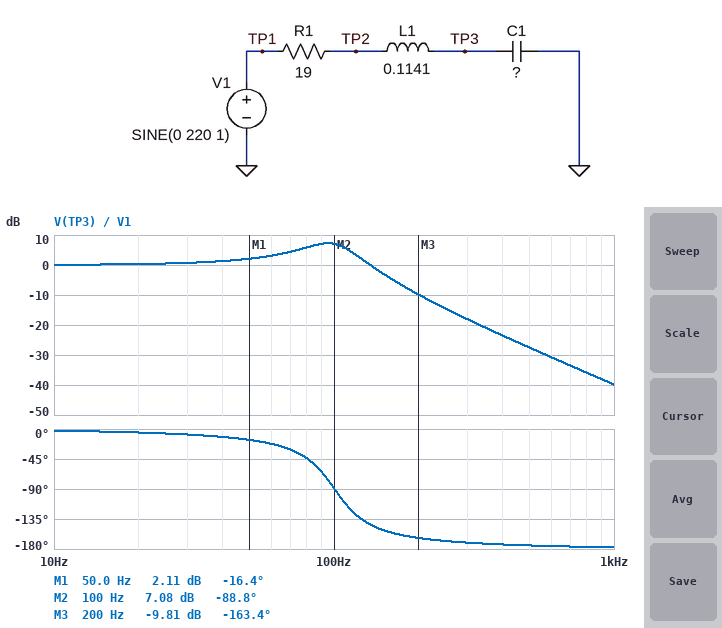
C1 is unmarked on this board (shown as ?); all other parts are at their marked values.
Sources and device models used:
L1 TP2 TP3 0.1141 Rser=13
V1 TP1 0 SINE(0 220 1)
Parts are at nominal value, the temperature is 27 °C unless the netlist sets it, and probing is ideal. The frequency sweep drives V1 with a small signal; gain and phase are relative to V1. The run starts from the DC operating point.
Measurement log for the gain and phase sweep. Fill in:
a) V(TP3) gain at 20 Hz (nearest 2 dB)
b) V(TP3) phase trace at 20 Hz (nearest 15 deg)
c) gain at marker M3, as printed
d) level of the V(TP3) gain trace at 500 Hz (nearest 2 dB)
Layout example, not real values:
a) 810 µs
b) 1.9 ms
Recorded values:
a) 0 dB
b) 0 deg
c) -9.81 dB
d) -28 dB
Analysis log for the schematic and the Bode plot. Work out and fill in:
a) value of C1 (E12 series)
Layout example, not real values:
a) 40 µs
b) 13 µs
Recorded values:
a) 22 µF
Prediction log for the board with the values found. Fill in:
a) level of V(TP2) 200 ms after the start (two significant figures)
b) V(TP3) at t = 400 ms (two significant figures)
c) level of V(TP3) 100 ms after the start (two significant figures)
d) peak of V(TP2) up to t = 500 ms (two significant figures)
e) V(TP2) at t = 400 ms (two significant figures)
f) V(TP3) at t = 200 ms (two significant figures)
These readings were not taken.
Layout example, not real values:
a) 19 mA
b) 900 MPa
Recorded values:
a) 210 V
b) 130 V
c) 130 V
d) 220 V
e) 130 V
f) 210 V
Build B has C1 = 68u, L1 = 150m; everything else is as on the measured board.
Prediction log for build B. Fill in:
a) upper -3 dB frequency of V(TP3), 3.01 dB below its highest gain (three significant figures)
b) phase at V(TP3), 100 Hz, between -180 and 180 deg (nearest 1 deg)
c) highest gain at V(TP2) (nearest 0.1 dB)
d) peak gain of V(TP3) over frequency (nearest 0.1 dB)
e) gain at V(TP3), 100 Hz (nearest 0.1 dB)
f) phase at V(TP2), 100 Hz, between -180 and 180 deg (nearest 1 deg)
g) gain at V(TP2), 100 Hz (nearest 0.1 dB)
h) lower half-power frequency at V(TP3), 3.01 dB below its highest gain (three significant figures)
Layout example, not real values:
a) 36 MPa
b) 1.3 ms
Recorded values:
a) 59.1 Hz
b) -156 deg
c) 0 dB
d) 3.9 dB
e) -10.4 dB
f) 14 deg
g) -0.7 dB
h) 17.8 Hz
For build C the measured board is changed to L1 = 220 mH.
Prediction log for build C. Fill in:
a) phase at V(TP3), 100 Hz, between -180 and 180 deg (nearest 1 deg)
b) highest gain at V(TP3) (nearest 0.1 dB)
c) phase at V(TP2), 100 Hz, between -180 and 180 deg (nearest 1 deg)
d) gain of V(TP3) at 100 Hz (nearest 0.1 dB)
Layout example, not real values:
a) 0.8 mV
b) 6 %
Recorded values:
a) -154 deg
b) 10.0 dB
c) 15 deg
d) -0.1 dB
